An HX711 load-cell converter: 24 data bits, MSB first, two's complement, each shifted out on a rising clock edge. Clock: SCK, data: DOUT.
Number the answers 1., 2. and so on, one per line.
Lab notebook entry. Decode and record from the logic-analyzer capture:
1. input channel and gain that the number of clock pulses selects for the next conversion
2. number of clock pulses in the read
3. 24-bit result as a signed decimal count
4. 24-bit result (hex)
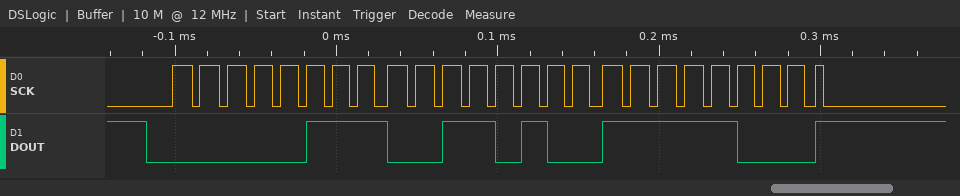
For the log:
1. channel A, gain 128
2. 25
3. 472312
4. 0x0734F8
